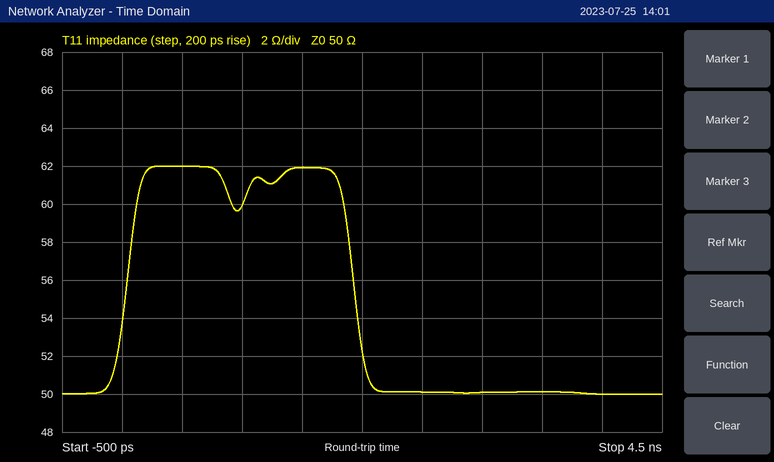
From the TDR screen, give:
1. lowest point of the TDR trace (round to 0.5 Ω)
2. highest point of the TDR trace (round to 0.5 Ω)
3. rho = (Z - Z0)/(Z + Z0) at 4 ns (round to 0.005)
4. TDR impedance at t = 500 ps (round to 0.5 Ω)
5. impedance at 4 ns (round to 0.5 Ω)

50.0 Ω
62.0 Ω
0.000
62.0 Ω
50.0 Ω
